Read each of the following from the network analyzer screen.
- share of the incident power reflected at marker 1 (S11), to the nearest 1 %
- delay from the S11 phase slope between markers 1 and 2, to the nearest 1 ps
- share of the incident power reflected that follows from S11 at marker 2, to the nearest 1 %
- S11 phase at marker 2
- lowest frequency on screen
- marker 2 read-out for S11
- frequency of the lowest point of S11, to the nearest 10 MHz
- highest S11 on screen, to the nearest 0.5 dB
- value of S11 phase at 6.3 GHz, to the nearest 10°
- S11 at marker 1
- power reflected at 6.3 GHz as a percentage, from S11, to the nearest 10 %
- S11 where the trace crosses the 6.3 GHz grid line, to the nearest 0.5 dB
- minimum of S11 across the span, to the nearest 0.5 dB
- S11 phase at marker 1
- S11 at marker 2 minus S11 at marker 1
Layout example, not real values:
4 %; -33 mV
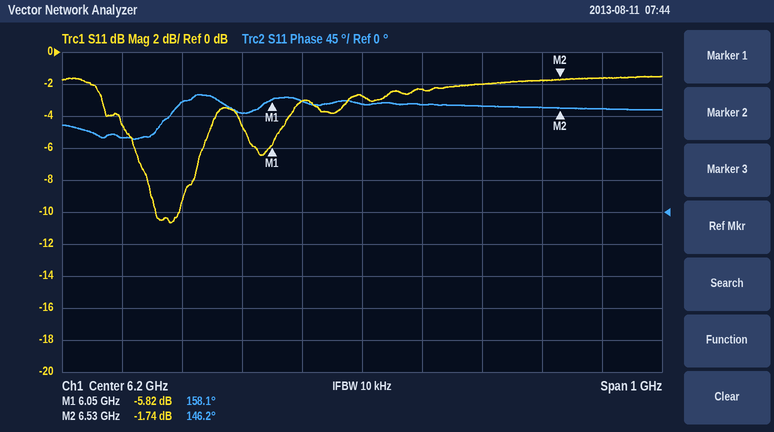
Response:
26 %; 69 ps; 67 %; 146.2°; 5.7 GHz; -1.74 dB; 5.88 GHz; -1.5 dB; 150°; -5.82 dB; 60 %; -2.5 dB; -10.5 dB; 158.1°; 4.08 dB
